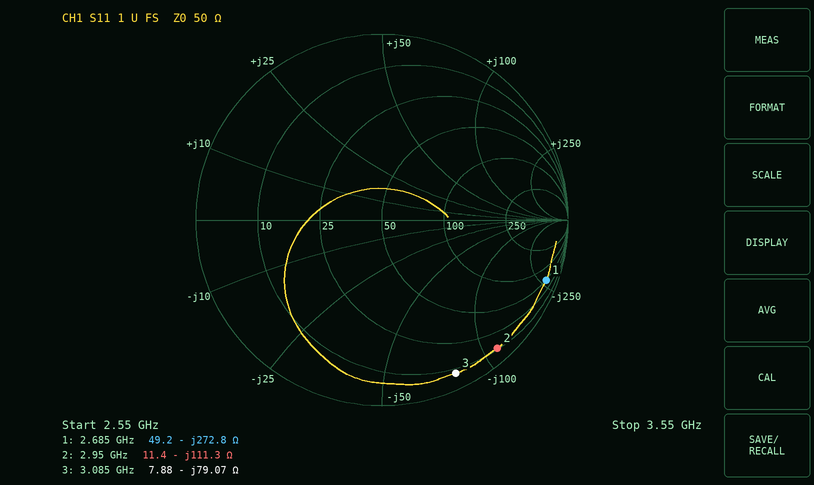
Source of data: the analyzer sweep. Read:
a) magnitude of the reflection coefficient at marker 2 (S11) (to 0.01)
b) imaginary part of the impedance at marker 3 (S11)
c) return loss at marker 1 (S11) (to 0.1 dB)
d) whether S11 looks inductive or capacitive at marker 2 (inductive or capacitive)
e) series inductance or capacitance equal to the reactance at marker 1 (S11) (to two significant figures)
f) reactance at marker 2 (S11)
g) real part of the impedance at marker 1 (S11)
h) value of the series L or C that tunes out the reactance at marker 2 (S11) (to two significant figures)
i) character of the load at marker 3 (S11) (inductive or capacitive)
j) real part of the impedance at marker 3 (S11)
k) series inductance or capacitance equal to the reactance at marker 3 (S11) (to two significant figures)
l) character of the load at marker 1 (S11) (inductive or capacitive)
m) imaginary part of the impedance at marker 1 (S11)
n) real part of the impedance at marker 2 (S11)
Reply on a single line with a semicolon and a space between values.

0.93; -79.07 Ω; 0.5 dB; capacitive; 220 fF; -111.3 Ω; 49.2 Ω; 6.0 nH; capacitive; 7.88 Ω; 650 fF; capacitive; -272.8 Ω; 11.4 Ω
